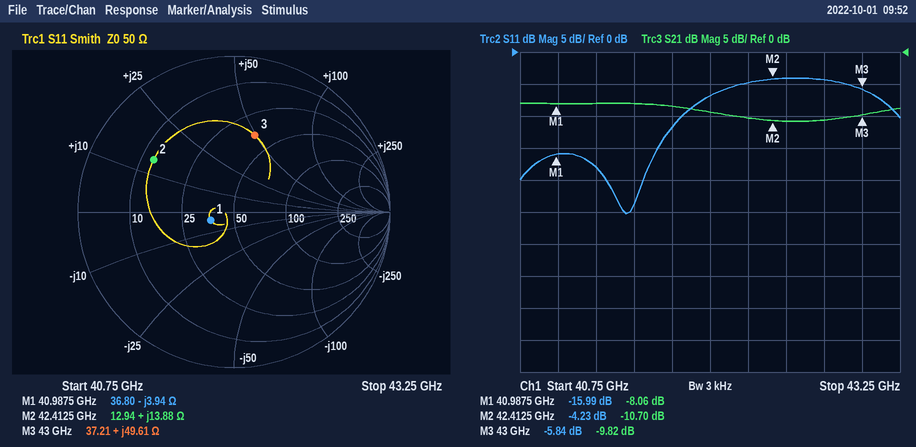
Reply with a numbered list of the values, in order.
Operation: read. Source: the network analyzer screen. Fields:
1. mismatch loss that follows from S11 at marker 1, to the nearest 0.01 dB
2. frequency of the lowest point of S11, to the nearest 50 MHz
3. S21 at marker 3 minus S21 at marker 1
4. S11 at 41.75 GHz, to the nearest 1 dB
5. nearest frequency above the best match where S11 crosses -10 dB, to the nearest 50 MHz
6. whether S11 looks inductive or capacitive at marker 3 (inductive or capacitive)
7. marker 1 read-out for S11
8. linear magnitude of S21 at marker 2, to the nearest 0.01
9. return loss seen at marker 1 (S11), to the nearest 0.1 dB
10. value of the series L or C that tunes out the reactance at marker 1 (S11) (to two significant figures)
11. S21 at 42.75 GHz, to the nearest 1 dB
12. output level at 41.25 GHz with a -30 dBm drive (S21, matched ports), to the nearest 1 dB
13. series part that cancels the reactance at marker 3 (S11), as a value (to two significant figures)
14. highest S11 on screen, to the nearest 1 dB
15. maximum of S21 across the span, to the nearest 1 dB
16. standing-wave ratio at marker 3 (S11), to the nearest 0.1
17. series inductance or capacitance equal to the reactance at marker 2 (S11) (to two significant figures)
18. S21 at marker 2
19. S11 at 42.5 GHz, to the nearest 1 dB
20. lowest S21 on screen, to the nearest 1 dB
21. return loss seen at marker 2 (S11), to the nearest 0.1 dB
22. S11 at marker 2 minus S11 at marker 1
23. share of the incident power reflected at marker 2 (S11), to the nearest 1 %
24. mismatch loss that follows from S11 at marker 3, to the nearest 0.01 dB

1. 0.11 dB
2. 41.45 GHz
3. -1.76 dB
4. -12 dB
5. 41.80 GHz
6. inductive
7. -15.99 dB
8. 0.29
9. 16.0 dB
10. 15 pH
11. -11 dB
12. -38 dBm
13. 75 fF
14. -4 dB
15. -8 dB
16. 3.1
17. 52 pH
18. -10.70 dB
19. -4 dB
20. -11 dB
21. 4.2 dB
22. 11.76 dB
23. 38 %
24. 1.31 dB
